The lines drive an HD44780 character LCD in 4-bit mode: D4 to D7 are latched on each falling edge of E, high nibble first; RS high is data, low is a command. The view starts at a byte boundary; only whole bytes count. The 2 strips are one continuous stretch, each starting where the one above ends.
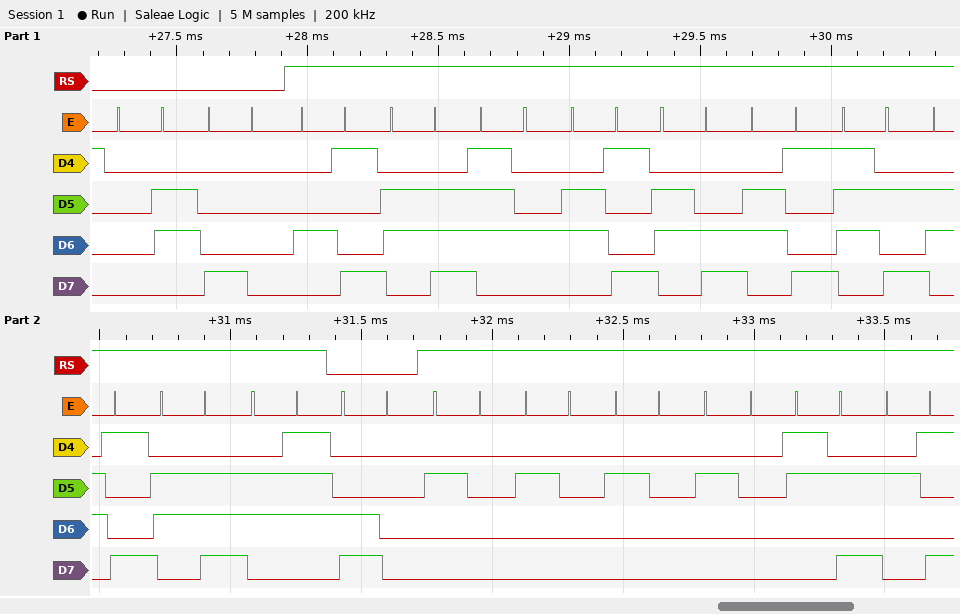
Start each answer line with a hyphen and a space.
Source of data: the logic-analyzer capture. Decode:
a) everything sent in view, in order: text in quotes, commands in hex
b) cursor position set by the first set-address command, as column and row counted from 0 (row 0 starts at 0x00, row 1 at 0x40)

- 0x06 0x80 "Intilizing" 0xC0 "    :)"
- column 0, row 0
